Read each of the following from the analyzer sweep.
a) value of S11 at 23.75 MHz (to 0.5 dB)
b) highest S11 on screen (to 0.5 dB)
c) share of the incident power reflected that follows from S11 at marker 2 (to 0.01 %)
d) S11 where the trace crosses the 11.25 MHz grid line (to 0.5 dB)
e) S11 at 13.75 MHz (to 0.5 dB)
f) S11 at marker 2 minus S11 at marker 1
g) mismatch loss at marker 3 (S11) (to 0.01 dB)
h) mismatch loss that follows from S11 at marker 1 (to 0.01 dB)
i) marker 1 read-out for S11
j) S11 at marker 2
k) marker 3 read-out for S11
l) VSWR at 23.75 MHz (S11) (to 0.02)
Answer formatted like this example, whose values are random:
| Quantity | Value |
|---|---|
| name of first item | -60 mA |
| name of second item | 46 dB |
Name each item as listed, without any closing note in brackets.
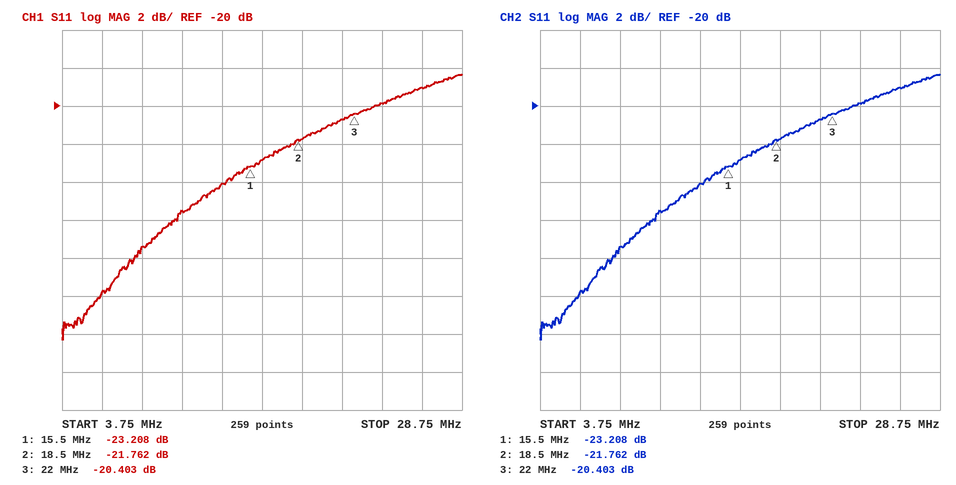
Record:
| Quantity | Value |
|---|---|
| value of S11 at 23.75 MHz | -20.0 dB |
| highest S11 on screen | -18.5 dB |
| share of the incident power reflected that follows from S11 at marker 2 | 0.67 % |
| S11 where the trace crosses the 11.25 MHz grid line | -25.5 dB |
| S11 at 13.75 MHz | -24.0 dB |
| S11 at marker 2 minus S11 at marker 1 | 1.446 dB |
| mismatch loss at marker 3 (S11) | 0.04 dB |
| mismatch loss that follows from S11 at marker 1 | 0.02 dB |
| marker 1 read-out for S11 | -23.208 dB |
| S11 at marker 2 | -21.762 dB |
| marker 3 read-out for S11 | -20.403 dB |
| VSWR at 23.75 MHz (S11) | 1.22 |
